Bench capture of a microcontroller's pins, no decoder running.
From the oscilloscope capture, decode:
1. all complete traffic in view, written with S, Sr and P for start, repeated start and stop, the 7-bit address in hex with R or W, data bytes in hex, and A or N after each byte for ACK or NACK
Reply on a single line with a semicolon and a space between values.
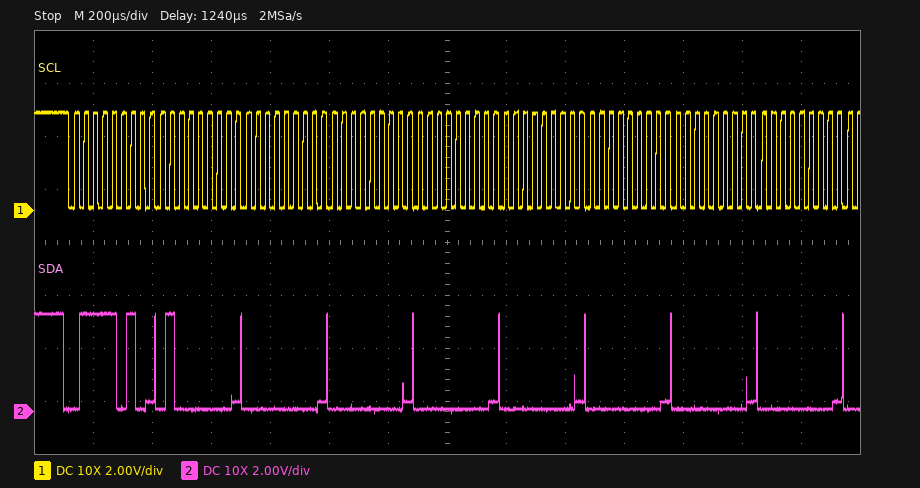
S 3DW A 40 A 00 A 00 A 00 A 00 A 00 A 00 A 00 A
